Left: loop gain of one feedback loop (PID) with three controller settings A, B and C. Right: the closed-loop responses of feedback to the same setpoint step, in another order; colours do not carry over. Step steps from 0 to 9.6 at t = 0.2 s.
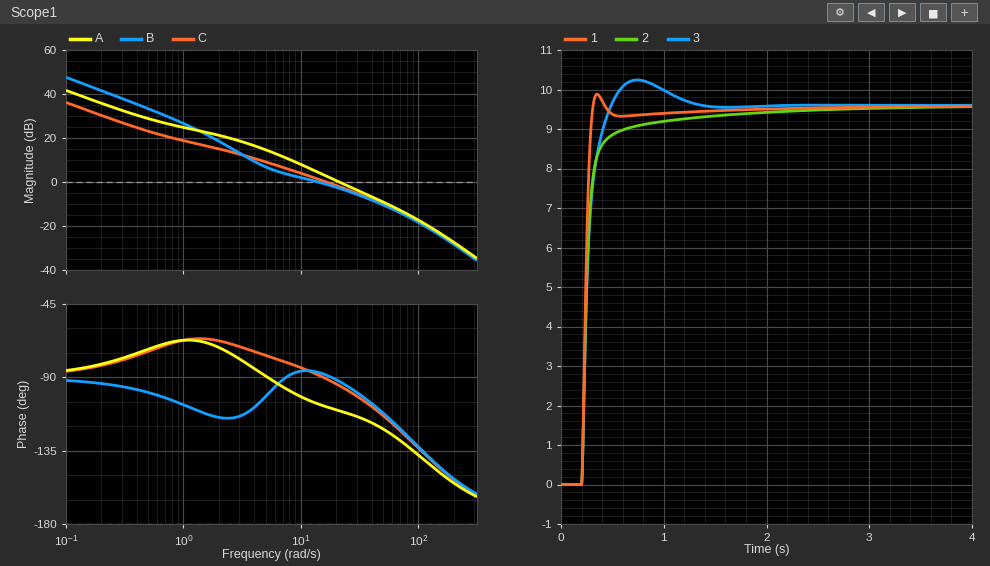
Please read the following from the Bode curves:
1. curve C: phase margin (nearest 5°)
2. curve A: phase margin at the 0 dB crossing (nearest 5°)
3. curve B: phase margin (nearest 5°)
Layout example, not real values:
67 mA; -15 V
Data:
90°; 70°; 95°
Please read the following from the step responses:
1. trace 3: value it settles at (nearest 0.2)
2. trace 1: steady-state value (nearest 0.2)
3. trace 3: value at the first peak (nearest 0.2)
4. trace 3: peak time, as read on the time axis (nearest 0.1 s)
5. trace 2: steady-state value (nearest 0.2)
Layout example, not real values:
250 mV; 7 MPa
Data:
9.6; 9.6; 10.2; 0.7 s; 9.6
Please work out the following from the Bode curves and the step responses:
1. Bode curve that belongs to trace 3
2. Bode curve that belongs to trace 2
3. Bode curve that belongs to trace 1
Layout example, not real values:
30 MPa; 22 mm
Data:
B; C; A
